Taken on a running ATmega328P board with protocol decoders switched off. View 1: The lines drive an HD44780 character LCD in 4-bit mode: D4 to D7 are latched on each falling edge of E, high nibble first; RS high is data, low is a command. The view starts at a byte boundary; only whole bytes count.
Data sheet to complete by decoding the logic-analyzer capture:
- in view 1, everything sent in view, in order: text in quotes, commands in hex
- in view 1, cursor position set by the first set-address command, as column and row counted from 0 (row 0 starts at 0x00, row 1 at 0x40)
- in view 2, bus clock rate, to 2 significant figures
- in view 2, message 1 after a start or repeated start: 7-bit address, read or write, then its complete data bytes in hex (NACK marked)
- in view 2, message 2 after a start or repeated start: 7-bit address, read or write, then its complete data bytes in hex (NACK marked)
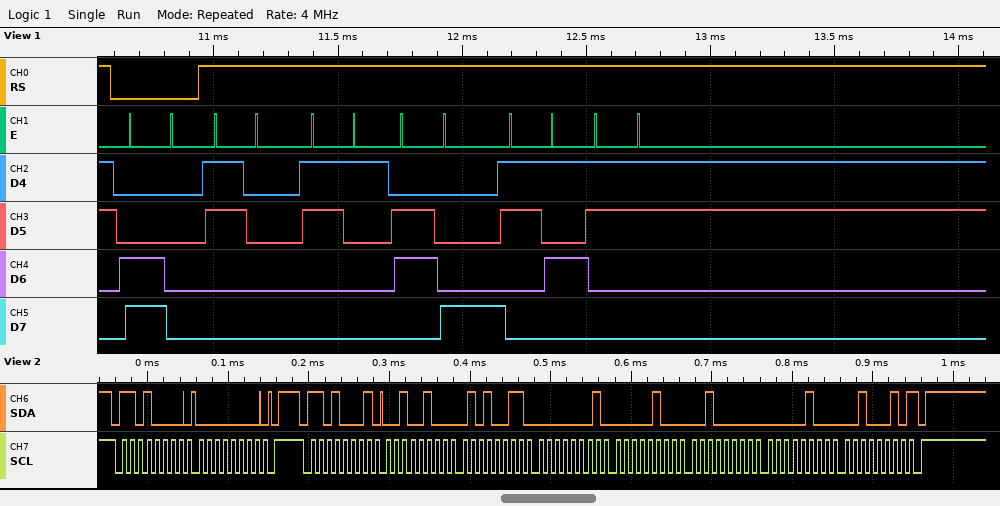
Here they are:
0xC0 "01h53"
column 0, row 1
100 kHz
0x68 write: 00
0x68 read: 24 53 01 04 20 04 22 NACK
